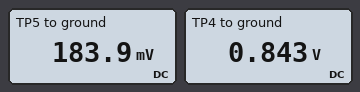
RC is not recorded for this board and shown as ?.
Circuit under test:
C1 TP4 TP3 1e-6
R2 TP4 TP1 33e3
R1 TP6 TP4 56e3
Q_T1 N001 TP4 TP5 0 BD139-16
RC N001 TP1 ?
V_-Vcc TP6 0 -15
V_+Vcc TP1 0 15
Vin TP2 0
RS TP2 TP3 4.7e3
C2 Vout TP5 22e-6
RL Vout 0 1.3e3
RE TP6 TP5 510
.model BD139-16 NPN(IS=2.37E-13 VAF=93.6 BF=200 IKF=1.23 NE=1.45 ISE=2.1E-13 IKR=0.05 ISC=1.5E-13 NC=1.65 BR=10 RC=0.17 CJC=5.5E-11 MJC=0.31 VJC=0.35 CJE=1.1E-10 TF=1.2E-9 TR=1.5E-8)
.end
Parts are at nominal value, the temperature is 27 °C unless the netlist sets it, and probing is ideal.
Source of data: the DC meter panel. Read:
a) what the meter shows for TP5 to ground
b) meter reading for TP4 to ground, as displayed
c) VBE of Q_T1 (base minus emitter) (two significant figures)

183.9 mV
0.843 V
660 mV
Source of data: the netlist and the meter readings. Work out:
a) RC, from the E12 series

150 Ω
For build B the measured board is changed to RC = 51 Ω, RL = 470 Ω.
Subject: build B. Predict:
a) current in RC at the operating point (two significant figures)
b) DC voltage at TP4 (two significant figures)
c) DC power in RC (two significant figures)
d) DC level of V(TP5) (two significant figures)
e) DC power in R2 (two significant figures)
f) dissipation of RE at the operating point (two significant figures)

30 mA
910 mV
45 mW
250 mV
6.0 mW
460 mW
